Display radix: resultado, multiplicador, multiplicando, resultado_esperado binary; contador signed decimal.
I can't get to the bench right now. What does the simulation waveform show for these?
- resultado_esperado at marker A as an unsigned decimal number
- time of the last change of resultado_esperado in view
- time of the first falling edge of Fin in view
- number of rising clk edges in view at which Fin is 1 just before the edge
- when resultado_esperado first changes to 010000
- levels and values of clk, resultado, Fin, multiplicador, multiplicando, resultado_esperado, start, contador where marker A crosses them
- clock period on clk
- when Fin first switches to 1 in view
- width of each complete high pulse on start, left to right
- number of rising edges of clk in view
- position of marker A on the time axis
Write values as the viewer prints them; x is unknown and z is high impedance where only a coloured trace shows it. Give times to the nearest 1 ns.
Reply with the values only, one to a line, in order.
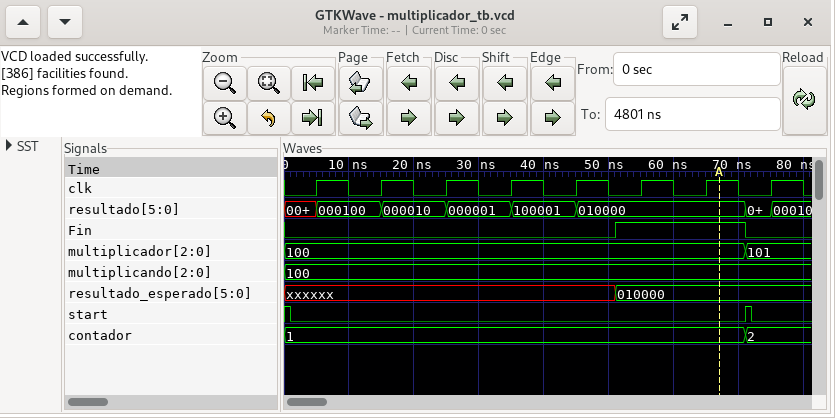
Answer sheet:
16
51 ns
71 ns
2
51 ns
clk=1, resultado=010000, Fin=1, multiplicador=100, multiplicando=100, resultado_esperado=010000, start=0, contador=1
10 ns
51 ns
1 ns
8
67 ns
